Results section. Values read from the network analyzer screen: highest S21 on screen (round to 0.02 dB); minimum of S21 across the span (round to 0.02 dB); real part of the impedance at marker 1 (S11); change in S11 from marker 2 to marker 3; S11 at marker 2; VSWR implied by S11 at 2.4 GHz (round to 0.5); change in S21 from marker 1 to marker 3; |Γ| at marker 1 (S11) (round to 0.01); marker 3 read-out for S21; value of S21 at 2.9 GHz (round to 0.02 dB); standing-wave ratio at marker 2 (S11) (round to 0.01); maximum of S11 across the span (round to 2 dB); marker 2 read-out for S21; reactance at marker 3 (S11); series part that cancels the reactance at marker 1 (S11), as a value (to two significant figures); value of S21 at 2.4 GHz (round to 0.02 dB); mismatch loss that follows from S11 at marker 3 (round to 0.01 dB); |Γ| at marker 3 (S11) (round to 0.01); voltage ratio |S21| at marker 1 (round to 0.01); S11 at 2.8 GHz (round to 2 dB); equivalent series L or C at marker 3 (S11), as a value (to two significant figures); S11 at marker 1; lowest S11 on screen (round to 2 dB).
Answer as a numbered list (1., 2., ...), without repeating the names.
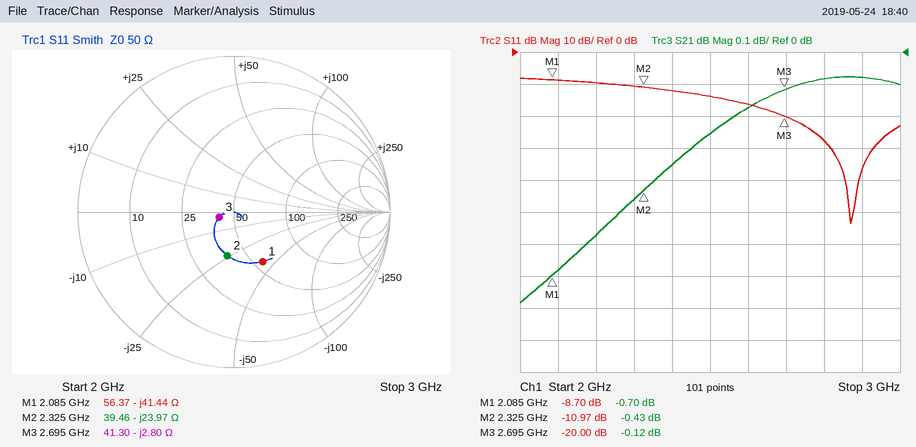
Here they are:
1. -0.08 dB
2. -0.78 dB
3. 56.37 Ω
4. -9.03 dB
5. -10.97 dB
6. 1.5
7. 0.58 dB
8. 0.37
9. -0.12 dB
10. -0.08 dB
11. 1.79
12. -8 dB
13. -0.43 dB
14. -2.80 Ω
15. 3.2 nH
16. -0.36 dB
17. 0.04 dB
18. 0.10
19. 0.92
20. -28 dB
21. 21 pF
22. -8.70 dB
23. -54 dB
